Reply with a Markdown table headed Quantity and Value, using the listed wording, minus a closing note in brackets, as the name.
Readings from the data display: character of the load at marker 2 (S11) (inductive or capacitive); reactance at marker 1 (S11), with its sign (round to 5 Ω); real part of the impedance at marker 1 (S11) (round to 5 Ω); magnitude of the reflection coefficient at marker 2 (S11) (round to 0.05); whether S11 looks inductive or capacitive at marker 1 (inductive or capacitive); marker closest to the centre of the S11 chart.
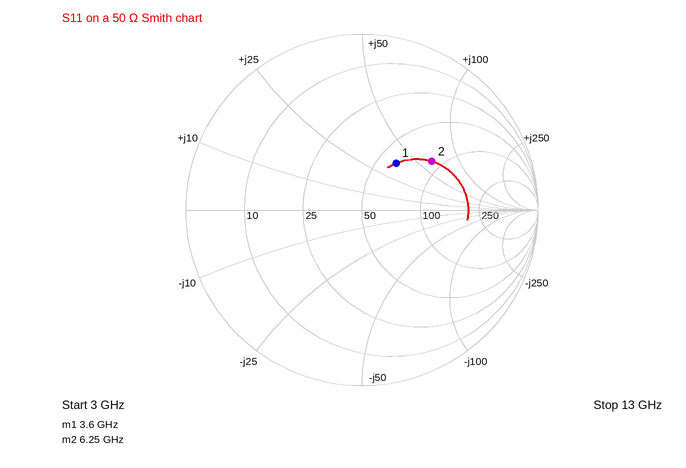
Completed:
| Quantity | Value |
|---|---|
| character of the load at marker 2 (S11) | inductive |
| reactance at marker 1 (S11), with its sign | +35 Ω |
| real part of the impedance at marker 1 (S11) | 60 Ω |
| magnitude of the reflection coefficient at marker 2 (S11) | 0.50 |
| whether S11 looks inductive or capacitive at marker 1 | inductive |
| marker closest to the centre of the S11 chart | marker 1 |
